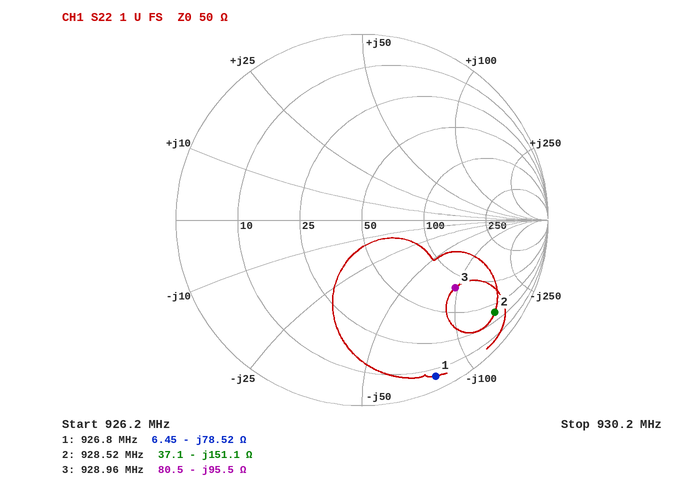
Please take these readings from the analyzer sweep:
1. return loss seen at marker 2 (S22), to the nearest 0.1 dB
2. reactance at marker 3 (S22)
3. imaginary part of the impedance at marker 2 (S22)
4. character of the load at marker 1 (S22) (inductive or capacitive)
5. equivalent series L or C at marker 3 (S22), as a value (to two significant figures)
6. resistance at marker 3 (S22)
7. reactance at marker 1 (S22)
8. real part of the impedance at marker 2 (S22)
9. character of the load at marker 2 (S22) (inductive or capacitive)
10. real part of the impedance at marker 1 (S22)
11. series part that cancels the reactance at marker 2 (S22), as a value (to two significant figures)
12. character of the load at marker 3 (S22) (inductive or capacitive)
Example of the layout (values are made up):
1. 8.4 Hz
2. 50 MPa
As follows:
1. 1.2 dB
2. -95.5 Ω
3. -151.1 Ω
4. capacitive
5. 1.8 pF
6. 80.5 Ω
7. -78.52 Ω
8. 37.1 Ω
9. capacitive
10. 6.45 Ω
11. 26 nH
12. capacitive
